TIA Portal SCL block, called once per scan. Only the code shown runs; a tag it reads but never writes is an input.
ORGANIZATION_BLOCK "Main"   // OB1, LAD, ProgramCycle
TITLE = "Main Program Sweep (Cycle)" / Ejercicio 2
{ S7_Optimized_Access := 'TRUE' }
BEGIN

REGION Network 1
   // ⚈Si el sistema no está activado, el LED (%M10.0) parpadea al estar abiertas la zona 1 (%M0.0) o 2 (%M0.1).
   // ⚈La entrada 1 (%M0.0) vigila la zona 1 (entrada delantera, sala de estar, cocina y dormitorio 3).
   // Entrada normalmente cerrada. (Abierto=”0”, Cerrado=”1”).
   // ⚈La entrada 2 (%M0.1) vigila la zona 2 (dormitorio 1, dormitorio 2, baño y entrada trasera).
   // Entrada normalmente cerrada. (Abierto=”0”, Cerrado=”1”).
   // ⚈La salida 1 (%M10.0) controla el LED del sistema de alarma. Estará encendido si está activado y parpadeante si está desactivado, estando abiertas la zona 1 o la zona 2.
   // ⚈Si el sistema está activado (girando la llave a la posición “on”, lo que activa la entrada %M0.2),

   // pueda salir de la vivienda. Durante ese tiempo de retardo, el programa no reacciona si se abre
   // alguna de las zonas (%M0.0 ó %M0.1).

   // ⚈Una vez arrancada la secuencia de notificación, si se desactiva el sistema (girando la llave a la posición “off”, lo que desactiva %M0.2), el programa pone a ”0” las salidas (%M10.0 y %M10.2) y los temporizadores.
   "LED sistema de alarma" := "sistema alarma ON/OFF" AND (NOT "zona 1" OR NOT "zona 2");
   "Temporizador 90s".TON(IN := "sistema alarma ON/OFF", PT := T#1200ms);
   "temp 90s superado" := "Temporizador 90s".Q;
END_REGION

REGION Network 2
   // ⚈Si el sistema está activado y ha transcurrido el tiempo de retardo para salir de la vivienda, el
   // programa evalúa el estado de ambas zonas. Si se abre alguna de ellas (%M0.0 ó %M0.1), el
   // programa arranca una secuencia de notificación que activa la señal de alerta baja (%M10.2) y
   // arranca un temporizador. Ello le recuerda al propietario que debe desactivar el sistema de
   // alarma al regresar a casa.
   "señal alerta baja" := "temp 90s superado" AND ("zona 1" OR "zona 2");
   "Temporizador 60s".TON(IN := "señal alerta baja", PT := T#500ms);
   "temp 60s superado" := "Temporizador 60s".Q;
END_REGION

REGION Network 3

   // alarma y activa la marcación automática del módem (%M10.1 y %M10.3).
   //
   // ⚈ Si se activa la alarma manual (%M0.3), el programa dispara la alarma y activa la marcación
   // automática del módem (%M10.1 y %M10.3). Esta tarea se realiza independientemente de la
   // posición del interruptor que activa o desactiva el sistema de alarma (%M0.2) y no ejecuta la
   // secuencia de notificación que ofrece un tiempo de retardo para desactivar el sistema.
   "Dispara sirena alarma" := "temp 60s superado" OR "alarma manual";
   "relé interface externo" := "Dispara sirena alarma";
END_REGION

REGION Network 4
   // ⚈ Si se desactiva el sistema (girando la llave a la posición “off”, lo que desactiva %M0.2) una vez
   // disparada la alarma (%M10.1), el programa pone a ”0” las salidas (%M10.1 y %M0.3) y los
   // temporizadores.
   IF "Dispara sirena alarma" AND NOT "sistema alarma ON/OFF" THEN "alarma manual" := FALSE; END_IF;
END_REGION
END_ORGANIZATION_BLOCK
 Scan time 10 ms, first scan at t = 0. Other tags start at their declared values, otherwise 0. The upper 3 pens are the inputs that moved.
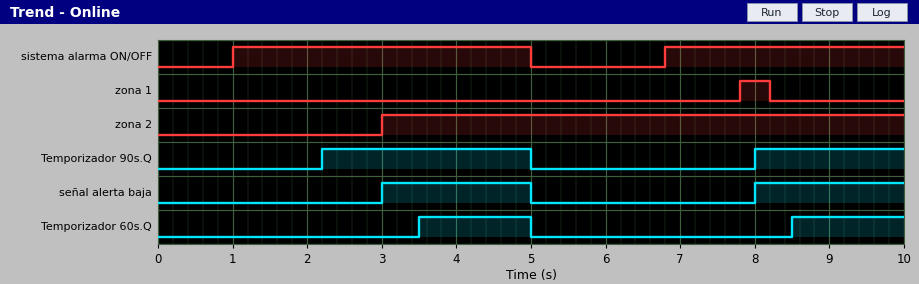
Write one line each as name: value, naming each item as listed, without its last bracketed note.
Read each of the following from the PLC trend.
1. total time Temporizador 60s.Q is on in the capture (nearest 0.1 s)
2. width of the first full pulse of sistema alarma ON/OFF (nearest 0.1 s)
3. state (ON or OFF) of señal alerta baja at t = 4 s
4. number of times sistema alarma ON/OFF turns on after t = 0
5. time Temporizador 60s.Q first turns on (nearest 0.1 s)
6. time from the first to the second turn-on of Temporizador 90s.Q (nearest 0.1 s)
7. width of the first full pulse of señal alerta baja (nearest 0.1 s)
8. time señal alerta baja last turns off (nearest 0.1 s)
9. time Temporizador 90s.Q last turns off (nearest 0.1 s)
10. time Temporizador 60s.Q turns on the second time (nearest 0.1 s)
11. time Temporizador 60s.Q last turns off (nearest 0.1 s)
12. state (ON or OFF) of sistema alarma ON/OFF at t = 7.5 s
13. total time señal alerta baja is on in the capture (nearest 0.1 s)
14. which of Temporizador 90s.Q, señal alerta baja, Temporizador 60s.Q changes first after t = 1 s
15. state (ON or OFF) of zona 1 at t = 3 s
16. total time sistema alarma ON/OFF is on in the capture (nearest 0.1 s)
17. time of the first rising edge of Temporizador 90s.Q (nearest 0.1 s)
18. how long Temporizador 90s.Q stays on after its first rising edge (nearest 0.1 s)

total time Temporizador 60s.Q is on in the capture: 3.0 s
width of the first full pulse of sistema alarma ON/OFF: 4.0 s
state (ON or OFF) of señal alerta baja at t = 4 s: ON
number of times sistema alarma ON/OFF turns on after t = 0: 2
time Temporizador 60s.Q first turns on: 3.5 s
time from the first to the second turn-on of Temporizador 90s.Q: 5.8 s
width of the first full pulse of señal alerta baja: 2.0 s
time señal alerta baja last turns off: 5.0 s
time Temporizador 90s.Q last turns off: 5.0 s
time Temporizador 60s.Q turns on the second time: 8.5 s
time Temporizador 60s.Q last turns off: 5.0 s
state (ON or OFF) of sistema alarma ON/OFF at t = 7.5 s: ON
total time señal alerta baja is on in the capture: 4.0 s
which of Temporizador 90s.Q, señal alerta baja, Temporizador 60s.Q changes first after t = 1 s: Temporizador 90s.Q
state (ON or OFF) of zona 1 at t = 3 s: OFF
total time sistema alarma ON/OFF is on in the capture: 7.2 s
time of the first rising edge of Temporizador 90s.Q: 2.2 s
how long Temporizador 90s.Q stays on after its first rising edge: 2.8 s
